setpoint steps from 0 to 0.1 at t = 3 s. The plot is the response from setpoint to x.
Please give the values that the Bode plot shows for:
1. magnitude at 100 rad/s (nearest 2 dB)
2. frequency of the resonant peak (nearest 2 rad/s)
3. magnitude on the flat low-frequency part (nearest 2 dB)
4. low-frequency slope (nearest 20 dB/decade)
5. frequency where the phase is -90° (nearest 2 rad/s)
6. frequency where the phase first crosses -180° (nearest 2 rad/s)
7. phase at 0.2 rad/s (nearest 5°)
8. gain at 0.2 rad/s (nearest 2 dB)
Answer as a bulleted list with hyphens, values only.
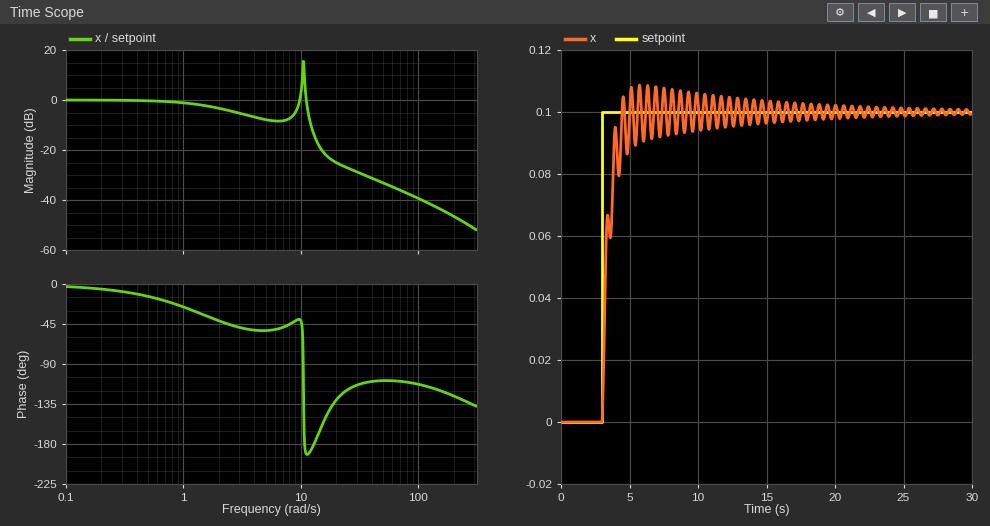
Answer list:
- -40 dB
- 10 rad/s
- 0 dB
- 0 dB/decade
- 10 rad/s
- 10 rad/s
- -5°
- 0 dB
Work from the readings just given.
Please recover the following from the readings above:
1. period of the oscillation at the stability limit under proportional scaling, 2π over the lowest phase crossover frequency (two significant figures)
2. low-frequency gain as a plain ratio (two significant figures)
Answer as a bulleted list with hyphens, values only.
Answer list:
- 0.63 s
- 1.0
